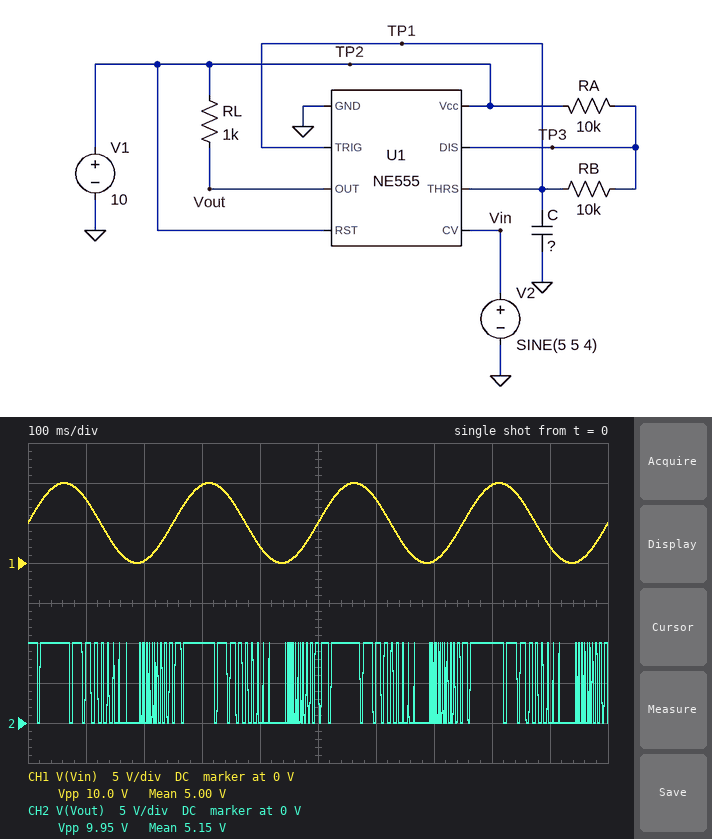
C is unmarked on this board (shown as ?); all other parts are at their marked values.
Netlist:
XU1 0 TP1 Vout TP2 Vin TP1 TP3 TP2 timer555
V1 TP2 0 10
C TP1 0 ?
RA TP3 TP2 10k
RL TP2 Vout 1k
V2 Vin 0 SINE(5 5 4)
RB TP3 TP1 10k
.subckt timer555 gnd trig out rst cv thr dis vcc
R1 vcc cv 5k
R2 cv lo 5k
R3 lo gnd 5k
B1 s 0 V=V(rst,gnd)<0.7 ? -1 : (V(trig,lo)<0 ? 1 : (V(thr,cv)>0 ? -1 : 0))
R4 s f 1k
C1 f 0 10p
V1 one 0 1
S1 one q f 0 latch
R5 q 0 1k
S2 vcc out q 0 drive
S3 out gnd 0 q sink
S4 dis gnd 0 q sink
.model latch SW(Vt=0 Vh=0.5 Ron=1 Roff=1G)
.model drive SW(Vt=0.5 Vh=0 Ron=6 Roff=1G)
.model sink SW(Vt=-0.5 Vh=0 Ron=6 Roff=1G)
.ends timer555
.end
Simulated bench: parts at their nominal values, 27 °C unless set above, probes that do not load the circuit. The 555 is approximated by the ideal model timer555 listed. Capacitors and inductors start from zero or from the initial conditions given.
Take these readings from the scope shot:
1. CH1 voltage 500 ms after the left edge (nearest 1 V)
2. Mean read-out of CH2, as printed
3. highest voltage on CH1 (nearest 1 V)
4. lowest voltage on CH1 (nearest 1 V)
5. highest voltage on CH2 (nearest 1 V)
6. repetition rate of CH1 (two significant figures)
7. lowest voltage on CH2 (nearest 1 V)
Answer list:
5 V
5.15 V
10 V
0 V
10 V
4.0 Hz
0 V
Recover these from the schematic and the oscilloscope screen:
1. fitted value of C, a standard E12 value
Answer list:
680 nF
